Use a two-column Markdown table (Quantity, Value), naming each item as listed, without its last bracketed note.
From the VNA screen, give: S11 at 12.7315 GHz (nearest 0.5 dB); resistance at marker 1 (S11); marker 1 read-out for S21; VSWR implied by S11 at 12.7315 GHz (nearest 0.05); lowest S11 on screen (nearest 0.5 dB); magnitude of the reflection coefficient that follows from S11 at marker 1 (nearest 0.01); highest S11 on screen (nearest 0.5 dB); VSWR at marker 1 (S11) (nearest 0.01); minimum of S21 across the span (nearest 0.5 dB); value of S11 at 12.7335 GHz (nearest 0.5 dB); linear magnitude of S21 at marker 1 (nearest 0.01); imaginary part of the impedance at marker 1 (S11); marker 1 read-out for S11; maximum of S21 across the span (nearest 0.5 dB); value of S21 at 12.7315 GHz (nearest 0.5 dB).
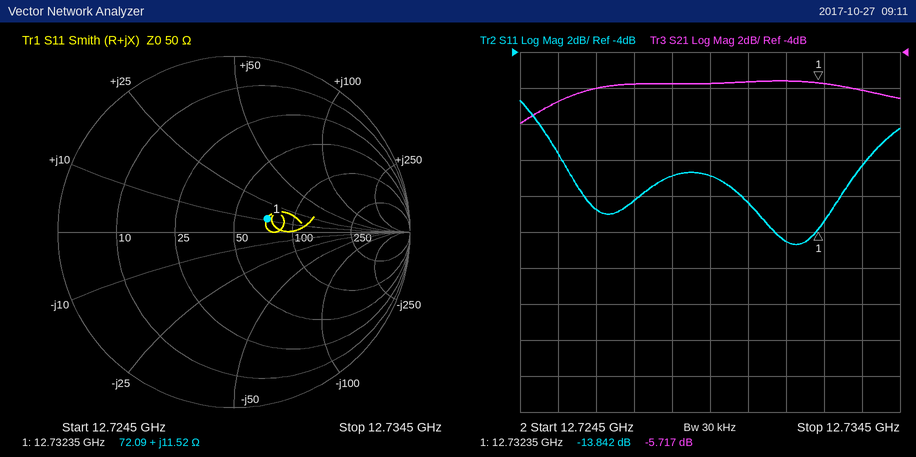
| Quantity | Value |
|---|---|
| S11 at 12.7315 GHz | -14.5 dB |
| resistance at marker 1 | 72.09 Ω |
| marker 1 read-out for S21 | -5.717 dB |
| VSWR implied by S11 at 12.7315 GHz | 1.45 |
| lowest S11 on screen | -14.5 dB |
| magnitude of the reflection coefficient that follows from S11 at marker 1 | 0.20 |
| highest S11 on screen | -6.5 dB |
| VSWR at marker 1 (S11) | 1.51 |
| minimum of S21 across the span | -8.0 dB |
| value of S11 at 12.7335 GHz | -10.5 dB |
| linear magnitude of S21 at marker 1 | 0.52 |
| imaginary part of the impedance at marker 1 | +11.52 Ω |
| marker 1 read-out for S11 | -13.842 dB |
| maximum of S21 across the span | -5.5 dB |
| value of S21 at 12.7315 GHz | -5.5 dB |
